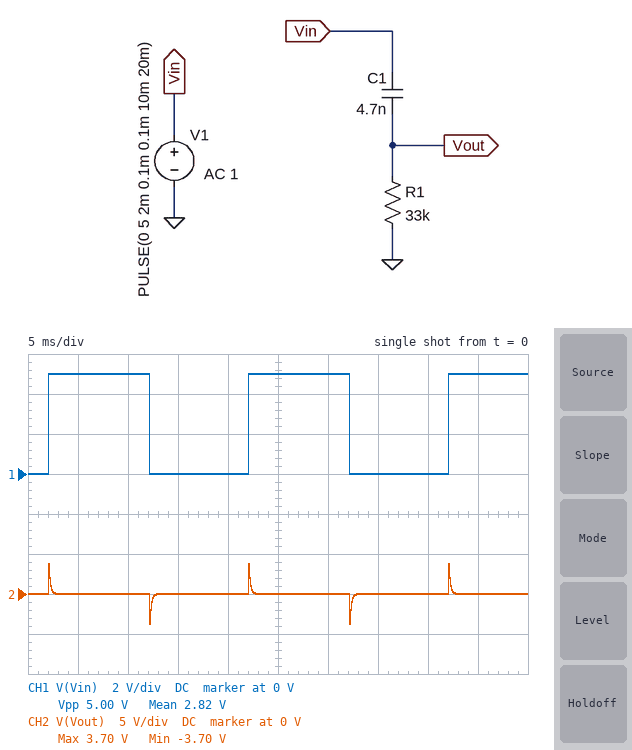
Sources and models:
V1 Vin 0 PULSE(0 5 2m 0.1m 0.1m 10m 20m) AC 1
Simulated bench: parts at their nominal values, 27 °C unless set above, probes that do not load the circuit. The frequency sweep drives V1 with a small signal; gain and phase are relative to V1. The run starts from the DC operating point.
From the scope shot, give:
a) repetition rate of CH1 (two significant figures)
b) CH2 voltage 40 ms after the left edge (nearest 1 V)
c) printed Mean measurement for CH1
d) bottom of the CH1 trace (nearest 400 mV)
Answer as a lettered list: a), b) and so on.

a) 50 Hz
b) 0 V
c) 2.82 V
d) 0 V
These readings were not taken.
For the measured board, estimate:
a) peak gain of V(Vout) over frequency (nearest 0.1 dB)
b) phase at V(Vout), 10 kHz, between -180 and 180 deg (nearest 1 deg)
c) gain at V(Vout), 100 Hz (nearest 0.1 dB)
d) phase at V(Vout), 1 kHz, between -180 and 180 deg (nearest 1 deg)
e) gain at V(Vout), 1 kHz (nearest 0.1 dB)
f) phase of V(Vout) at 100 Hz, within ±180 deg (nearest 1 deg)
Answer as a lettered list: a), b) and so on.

a) 0 dB
b) 6 deg
c) -20.3 dB
d) 46 deg
e) -3.1 dB
f) 84 deg
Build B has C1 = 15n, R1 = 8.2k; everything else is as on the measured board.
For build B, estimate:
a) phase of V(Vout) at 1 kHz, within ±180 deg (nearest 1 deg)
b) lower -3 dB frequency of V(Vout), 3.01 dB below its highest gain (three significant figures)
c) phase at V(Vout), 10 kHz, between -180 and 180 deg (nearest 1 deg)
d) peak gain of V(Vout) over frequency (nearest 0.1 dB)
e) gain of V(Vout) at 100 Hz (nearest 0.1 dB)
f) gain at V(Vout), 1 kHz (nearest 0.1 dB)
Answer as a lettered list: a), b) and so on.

a) 52 deg
b) 1.29 kHz
c) 7 deg
d) 0 dB
e) -22.3 dB
f) -4.3 dB
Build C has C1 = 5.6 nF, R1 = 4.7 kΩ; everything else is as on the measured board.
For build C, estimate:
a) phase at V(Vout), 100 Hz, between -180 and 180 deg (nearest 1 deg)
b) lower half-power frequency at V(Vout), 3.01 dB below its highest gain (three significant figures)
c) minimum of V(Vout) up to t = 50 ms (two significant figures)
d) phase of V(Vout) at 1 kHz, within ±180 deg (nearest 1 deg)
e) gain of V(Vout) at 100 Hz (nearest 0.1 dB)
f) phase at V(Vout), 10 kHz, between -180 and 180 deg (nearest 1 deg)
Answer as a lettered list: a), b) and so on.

a) 89 deg
b) 6.05 kHz
c) -1.3 V
d) 81 deg
e) -35.6 dB
f) 31 deg
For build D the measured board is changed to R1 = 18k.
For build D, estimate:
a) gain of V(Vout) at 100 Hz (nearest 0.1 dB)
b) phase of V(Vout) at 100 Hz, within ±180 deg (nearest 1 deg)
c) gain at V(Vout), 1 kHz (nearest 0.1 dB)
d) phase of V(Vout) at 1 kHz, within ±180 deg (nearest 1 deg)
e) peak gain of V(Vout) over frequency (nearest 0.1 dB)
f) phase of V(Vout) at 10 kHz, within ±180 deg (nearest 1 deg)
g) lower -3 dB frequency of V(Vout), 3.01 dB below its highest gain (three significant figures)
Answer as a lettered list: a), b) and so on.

a) -25.5 dB
b) 87 deg
c) -6.6 dB
d) 62 deg
e) 0 dB
f) 11 deg
g) 1.88 kHz
